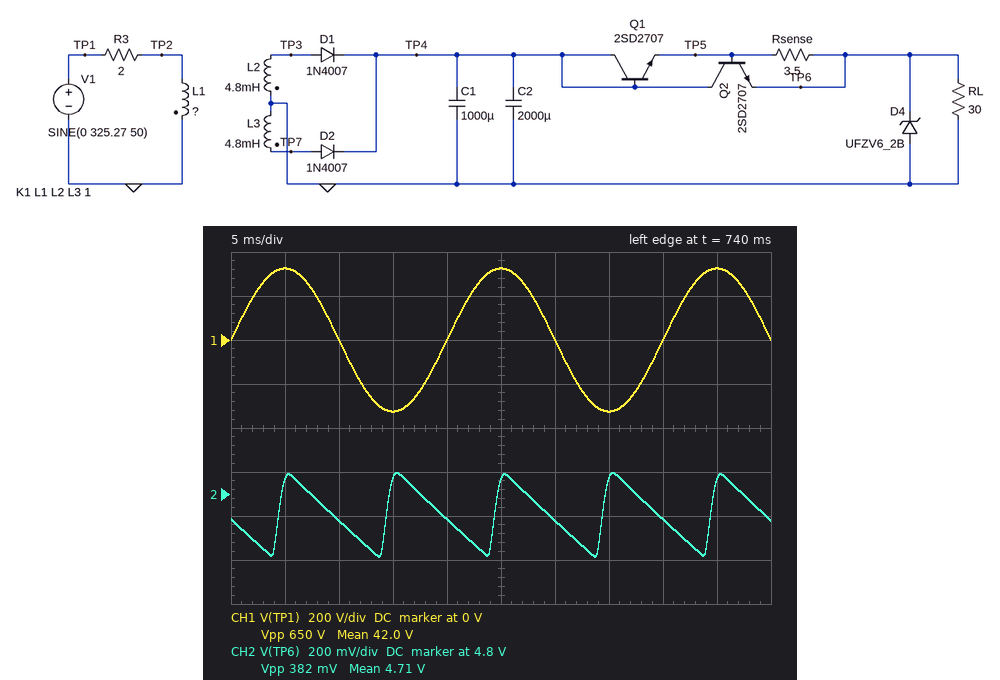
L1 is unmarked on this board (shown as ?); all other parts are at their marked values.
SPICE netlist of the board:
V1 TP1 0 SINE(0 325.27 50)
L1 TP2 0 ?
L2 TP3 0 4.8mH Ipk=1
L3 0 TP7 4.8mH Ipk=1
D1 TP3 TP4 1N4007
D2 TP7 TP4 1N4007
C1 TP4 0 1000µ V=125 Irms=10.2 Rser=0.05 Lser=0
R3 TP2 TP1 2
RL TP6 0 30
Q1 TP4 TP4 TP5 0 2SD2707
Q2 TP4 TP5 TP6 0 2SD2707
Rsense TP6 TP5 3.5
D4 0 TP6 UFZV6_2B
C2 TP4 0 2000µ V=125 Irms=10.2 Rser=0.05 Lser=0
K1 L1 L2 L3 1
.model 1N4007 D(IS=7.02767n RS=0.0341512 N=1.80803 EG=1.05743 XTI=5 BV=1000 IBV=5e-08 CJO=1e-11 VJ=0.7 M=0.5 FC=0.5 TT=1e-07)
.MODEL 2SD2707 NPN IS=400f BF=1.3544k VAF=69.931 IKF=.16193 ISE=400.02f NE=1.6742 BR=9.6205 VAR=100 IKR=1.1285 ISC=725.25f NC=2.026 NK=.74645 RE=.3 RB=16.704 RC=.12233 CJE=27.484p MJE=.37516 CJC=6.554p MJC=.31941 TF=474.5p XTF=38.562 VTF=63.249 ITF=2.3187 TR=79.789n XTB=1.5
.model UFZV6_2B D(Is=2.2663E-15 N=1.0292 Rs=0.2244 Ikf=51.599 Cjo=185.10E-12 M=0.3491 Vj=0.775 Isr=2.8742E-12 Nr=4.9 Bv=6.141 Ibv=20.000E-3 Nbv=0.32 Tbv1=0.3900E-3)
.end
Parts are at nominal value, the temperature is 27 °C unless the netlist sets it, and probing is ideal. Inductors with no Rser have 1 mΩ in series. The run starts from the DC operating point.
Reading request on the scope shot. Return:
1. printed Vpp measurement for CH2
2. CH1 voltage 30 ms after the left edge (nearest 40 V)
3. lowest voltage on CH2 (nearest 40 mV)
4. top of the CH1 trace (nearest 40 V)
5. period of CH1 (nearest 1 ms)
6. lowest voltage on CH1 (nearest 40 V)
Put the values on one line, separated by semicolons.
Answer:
382 mV; 0 V; 4.52 V; 320 V; 20 ms; -320 V
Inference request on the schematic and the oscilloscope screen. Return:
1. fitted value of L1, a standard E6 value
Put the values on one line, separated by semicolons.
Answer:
10 H
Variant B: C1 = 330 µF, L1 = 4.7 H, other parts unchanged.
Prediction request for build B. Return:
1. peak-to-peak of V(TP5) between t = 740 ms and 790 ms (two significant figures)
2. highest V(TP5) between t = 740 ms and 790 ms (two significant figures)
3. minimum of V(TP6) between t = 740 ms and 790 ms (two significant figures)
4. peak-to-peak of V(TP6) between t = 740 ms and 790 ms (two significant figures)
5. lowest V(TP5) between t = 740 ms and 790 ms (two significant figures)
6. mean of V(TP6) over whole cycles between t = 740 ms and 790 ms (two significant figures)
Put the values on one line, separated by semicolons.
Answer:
1.2 V; 8.0 V; 6.1 V; 220 mV; 6.8 V; 6.3 V
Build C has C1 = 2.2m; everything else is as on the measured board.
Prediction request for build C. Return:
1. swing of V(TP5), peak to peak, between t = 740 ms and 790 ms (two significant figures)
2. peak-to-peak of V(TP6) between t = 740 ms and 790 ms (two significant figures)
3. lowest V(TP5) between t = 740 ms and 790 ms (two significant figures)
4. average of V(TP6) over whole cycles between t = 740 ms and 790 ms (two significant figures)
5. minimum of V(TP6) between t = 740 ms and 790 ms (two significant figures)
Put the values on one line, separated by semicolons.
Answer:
310 mV; 280 mV; 5.1 V; 4.7 V; 4.6 V
